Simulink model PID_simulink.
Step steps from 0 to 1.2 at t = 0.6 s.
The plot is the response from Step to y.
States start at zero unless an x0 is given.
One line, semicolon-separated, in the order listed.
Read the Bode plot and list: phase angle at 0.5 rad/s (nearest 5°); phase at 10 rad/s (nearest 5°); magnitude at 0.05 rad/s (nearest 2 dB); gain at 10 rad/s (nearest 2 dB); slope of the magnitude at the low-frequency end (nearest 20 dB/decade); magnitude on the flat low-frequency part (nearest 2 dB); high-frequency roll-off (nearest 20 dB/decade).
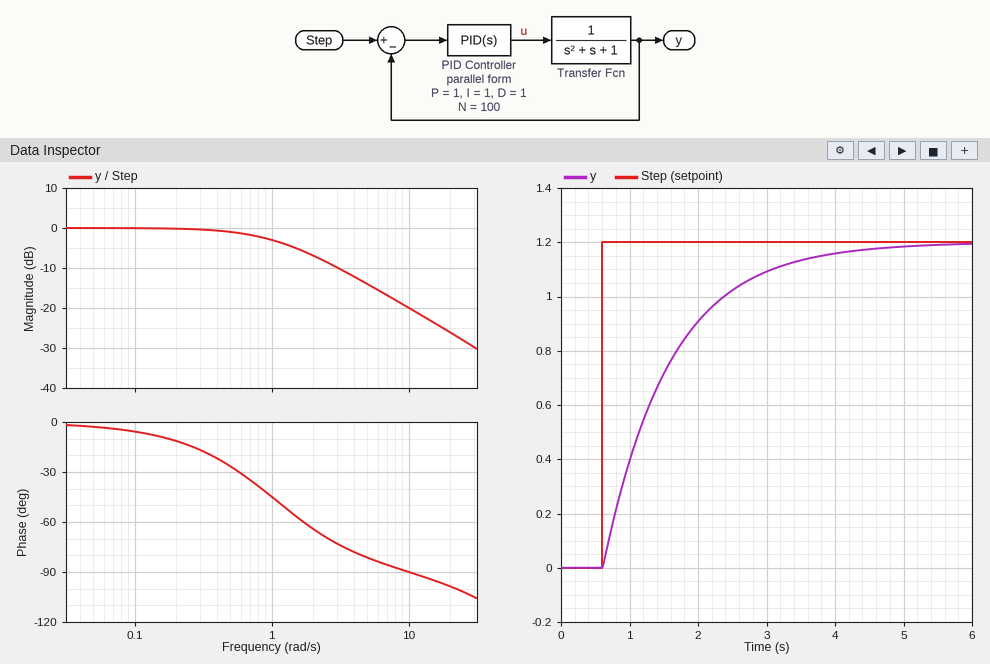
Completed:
-25°; -90°; 0 dB; -20 dB; 0 dB/decade; 0 dB; -20 dB/decade
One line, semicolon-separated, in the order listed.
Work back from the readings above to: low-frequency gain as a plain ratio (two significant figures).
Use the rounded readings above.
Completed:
1.0
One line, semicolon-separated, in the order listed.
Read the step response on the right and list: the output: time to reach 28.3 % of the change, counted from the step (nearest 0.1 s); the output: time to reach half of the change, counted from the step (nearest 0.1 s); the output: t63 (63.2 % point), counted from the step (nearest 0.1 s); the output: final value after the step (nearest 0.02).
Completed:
0.3 s; 0.7 s; 1.0 s; 1.20
